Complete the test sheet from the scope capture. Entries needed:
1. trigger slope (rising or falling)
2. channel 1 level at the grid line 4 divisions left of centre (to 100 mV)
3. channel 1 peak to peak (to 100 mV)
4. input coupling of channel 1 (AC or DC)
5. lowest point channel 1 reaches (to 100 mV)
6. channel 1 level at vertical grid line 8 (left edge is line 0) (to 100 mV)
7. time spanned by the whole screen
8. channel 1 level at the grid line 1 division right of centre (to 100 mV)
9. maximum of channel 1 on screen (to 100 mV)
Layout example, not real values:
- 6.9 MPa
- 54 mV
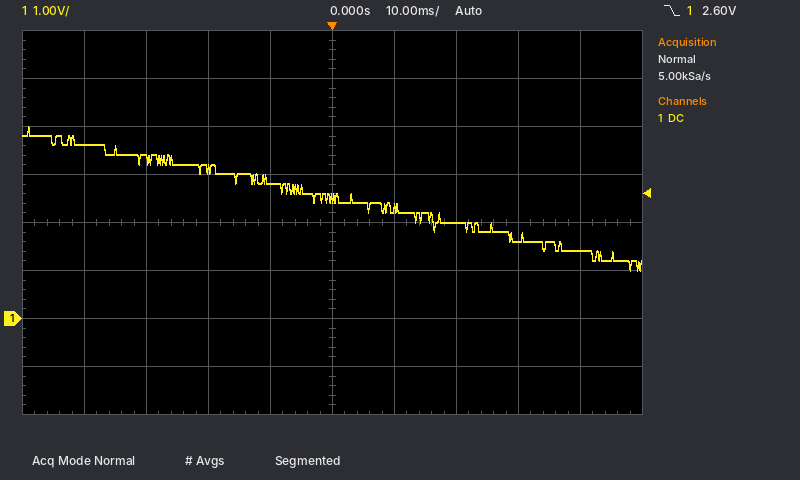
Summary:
- falling
- 3.6 V
- 3.0 V
- DC
- 1.0 V
- 1.6 V
- 100 ms
- 2.3 V
- 4.0 V
